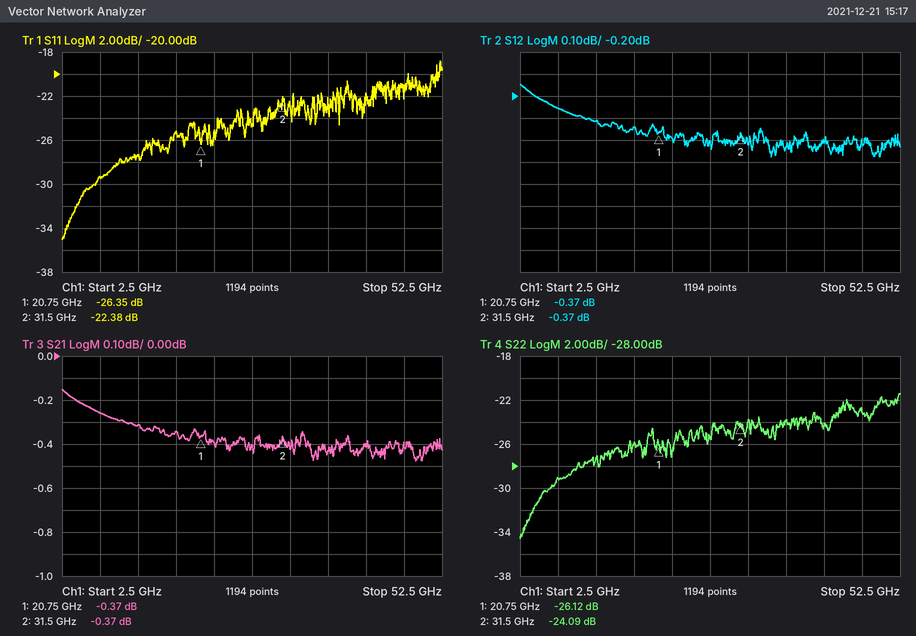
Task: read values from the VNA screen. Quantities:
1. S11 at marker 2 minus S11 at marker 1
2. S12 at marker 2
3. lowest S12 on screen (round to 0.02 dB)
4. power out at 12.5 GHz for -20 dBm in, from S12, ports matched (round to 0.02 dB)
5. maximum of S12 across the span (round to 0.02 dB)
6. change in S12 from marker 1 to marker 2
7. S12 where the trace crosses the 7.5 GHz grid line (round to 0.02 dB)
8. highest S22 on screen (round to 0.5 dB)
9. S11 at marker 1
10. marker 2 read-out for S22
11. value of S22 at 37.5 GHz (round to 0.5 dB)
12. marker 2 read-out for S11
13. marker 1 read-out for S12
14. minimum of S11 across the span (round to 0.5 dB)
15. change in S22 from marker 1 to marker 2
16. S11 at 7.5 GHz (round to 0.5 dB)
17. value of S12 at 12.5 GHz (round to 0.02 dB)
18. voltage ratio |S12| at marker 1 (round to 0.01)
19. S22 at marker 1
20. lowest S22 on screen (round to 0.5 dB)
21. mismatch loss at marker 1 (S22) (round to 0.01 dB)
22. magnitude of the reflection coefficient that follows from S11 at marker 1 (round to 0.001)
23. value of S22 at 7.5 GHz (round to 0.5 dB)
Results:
3.97 dB
-0.37 dB
-0.48 dB
-20.32 dBm
-0.14 dB
0.00 dB
-0.26 dB
-21.5 dB
-26.35 dB
-24.09 dB
-24.0 dB
-22.38 dB
-0.37 dB
-35.0 dB
2.03 dB
-29.5 dB
-0.32 dB
0.96
-26.12 dB
-34.5 dB
0.01 dB
0.048
-29.0 dB
